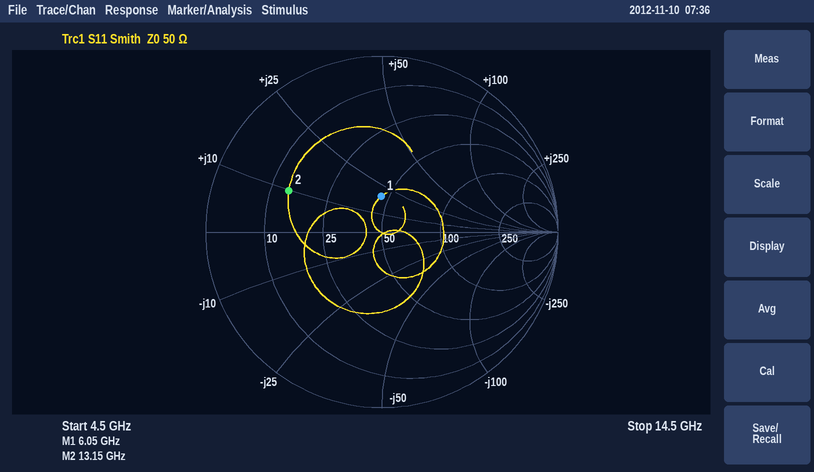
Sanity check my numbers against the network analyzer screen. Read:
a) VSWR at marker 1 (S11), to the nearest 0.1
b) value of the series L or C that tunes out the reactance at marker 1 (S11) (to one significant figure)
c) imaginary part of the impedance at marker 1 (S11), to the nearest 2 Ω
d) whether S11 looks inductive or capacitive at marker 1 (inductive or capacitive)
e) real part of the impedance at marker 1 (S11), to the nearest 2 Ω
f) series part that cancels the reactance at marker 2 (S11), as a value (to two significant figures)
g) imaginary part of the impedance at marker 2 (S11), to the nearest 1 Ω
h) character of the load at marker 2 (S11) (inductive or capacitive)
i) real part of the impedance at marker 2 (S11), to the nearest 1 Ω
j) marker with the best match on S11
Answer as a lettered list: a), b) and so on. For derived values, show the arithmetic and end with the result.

a) 1.5
b) C = 1/(2π × 6.05 GHz × 20 Ω) ≈ 1 pF
c) +20 Ω
d) inductive
e) 46 Ω
f) C = 1/(2π × 13.15 GHz × 10 Ω) ≈ 1.2 pF
g) +10 Ω
h) inductive
i) 14 Ω
j) marker 1
